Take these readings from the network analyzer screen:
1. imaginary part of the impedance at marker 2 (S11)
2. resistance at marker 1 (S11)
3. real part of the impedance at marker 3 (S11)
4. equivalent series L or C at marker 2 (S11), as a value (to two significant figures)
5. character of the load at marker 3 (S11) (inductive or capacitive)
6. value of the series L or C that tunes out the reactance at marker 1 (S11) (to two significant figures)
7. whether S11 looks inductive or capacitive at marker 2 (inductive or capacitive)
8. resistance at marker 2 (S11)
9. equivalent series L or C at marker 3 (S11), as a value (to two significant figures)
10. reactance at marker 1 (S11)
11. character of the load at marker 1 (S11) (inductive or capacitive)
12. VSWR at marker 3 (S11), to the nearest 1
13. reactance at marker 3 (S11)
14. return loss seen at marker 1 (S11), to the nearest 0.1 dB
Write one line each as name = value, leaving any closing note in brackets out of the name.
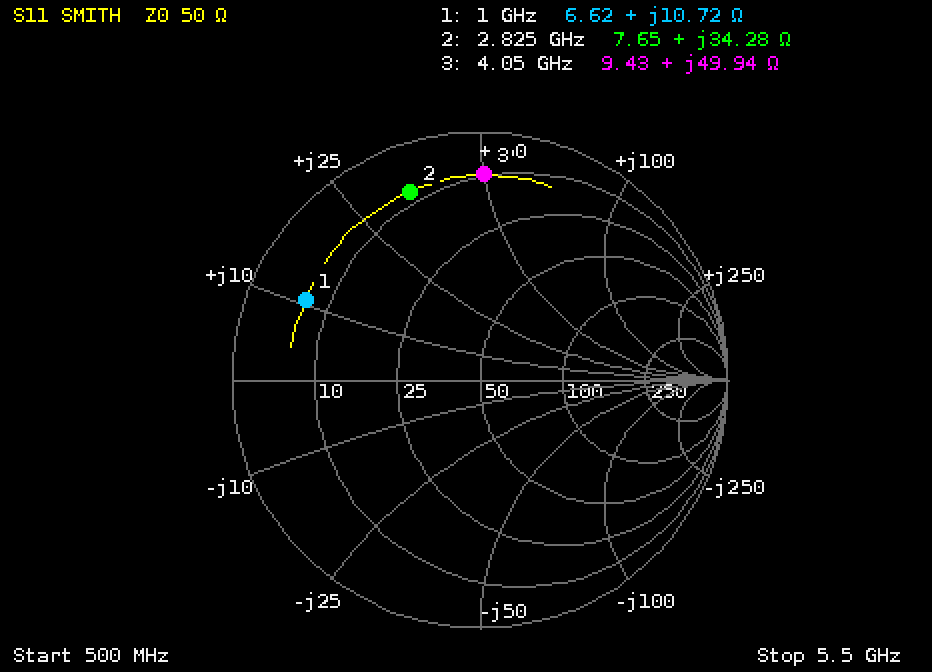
imaginary part of the impedance at marker 2 = +34.28 Ω
resistance at marker 1 = 6.62 Ω
real part of the impedance at marker 3 = 9.43 Ω
equivalent series L or C at marker 2 (S11), as a value = 1.9 nH
character of the load at marker 3 (S11) = inductive
value of the series L or C that tunes out the reactance at marker 1 (S11) = 15 pF
whether S11 looks inductive or capacitive at marker 2 = inductive
resistance at marker 2 = 7.65 Ω
equivalent series L or C at marker 3 (S11), as a value = 2.0 nH
reactance at marker 1 = +10.72 Ω
character of the load at marker 1 (S11) = inductive
VSWR at marker 3 (S11), to the nearest 1 = 11
reactance at marker 3 = +49.94 Ω
return loss seen at marker 1 (S11), to the nearest 0.1 dB = 2.2 dB
